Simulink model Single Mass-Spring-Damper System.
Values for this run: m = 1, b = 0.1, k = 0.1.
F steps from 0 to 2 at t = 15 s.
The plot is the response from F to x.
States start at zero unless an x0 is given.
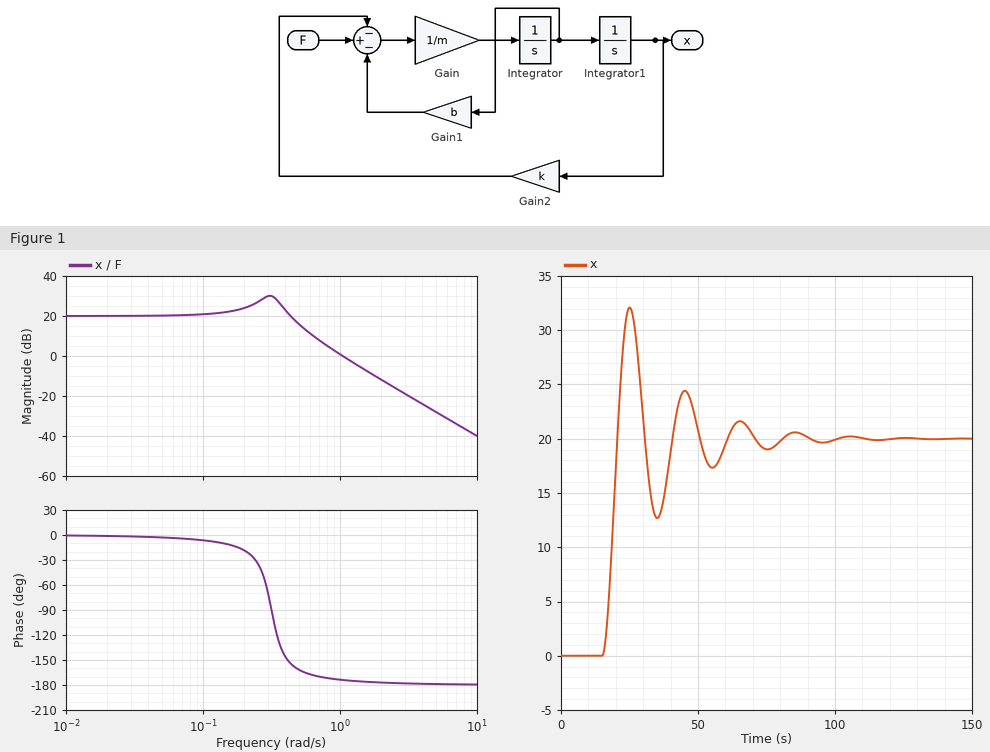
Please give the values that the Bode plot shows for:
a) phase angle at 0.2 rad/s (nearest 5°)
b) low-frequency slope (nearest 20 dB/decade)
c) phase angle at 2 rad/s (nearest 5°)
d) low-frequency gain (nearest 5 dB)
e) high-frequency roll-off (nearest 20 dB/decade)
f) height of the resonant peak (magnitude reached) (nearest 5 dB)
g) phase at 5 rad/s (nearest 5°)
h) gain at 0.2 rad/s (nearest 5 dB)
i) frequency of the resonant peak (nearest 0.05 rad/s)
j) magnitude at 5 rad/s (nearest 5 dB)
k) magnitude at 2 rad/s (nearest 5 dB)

-20°
0 dB/decade
-175°
20 dB
-40 dB/decade
30 dB
-180°
25 dB
0.30 rad/s
-30 dB
-10 dB
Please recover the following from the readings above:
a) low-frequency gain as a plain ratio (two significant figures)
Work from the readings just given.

10
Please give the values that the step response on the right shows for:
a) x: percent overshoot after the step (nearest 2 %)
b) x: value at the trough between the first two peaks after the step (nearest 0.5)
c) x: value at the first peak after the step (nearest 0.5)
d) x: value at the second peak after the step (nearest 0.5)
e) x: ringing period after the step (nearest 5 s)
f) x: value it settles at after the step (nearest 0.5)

60 %
12.5
32.0
24.5
20 s
20.0
